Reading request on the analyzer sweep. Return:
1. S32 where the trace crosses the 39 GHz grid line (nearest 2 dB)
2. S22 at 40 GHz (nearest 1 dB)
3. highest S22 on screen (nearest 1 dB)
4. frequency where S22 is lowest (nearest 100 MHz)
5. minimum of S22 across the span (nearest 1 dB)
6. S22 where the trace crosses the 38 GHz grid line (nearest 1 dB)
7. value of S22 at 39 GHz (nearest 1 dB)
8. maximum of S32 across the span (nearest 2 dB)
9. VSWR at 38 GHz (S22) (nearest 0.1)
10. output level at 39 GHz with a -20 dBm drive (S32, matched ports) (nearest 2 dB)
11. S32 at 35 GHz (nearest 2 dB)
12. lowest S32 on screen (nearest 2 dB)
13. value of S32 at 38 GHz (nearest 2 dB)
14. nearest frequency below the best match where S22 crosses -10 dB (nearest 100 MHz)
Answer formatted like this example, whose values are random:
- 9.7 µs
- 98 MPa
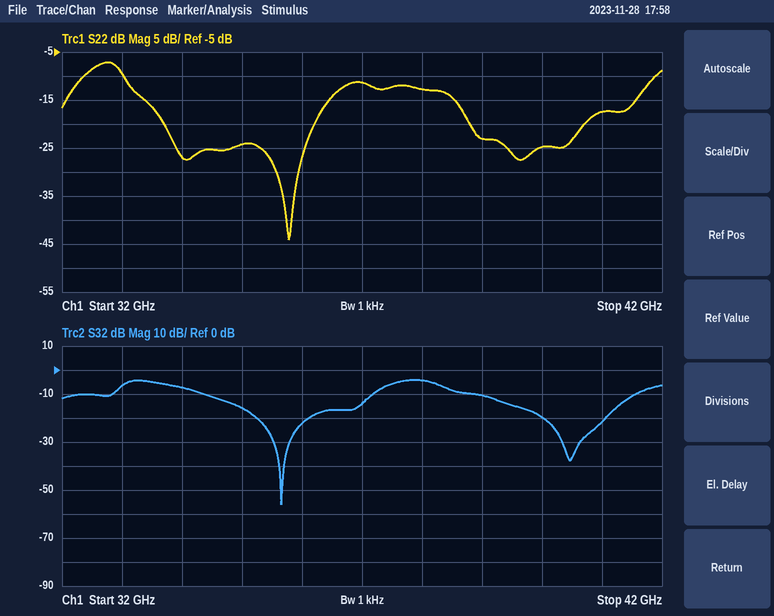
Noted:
- -10 dB
- -25 dB
- -7 dB
- 35.8 GHz
- -44 dB
- -13 dB
- -23 dB
- -4 dB
- 1.6
- -30 dBm
- -16 dB
- -56 dB
- -4 dB
- 33.0 GHz
